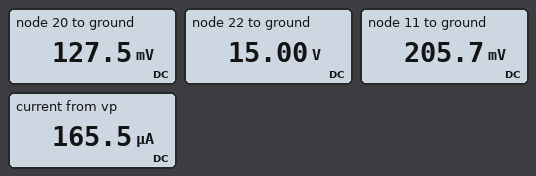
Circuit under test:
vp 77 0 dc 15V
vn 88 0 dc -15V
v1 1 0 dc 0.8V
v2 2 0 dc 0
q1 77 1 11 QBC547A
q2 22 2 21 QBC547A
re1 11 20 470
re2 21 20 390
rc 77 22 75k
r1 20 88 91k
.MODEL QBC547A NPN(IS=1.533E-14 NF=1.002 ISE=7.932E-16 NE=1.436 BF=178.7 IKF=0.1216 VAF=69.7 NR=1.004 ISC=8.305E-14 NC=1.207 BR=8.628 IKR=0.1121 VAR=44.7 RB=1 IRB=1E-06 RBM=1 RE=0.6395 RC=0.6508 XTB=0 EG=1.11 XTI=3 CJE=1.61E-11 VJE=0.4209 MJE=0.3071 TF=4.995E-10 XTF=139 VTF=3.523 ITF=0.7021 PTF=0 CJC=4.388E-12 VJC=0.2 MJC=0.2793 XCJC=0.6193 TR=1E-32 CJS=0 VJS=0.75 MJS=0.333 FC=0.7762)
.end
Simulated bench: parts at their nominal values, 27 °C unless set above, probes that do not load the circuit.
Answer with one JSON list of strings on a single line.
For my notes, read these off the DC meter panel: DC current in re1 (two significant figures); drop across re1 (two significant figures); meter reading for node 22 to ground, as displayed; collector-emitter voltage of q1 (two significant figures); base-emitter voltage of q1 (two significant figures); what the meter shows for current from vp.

["170 µA", "78 mV", "15.00 V", "15 V", "590 mV", "165.5 µA"]
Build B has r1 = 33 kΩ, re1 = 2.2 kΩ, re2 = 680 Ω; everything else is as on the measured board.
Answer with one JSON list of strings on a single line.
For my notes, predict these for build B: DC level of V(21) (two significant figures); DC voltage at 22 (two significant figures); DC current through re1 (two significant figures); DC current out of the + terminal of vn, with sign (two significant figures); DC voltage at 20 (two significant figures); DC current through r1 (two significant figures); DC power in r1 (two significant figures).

["-570 mV", "9.8 V", "370 µA", "-440 µA", "-620 mV", "440 µA", "6.3 mW"]
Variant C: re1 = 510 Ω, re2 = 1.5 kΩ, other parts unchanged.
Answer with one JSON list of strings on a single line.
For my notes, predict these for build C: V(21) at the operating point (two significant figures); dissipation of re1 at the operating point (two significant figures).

["120 mV", "14 µW"]
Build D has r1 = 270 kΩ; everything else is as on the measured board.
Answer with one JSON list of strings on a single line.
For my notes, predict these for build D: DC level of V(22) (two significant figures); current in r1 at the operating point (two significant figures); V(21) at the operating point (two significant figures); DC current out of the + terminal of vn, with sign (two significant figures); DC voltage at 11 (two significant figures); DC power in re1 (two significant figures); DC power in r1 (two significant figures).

["15 V", "56 µA", "210 mV", "-56 µA", "230 mV", "1.5 µW", "860 µW"]
